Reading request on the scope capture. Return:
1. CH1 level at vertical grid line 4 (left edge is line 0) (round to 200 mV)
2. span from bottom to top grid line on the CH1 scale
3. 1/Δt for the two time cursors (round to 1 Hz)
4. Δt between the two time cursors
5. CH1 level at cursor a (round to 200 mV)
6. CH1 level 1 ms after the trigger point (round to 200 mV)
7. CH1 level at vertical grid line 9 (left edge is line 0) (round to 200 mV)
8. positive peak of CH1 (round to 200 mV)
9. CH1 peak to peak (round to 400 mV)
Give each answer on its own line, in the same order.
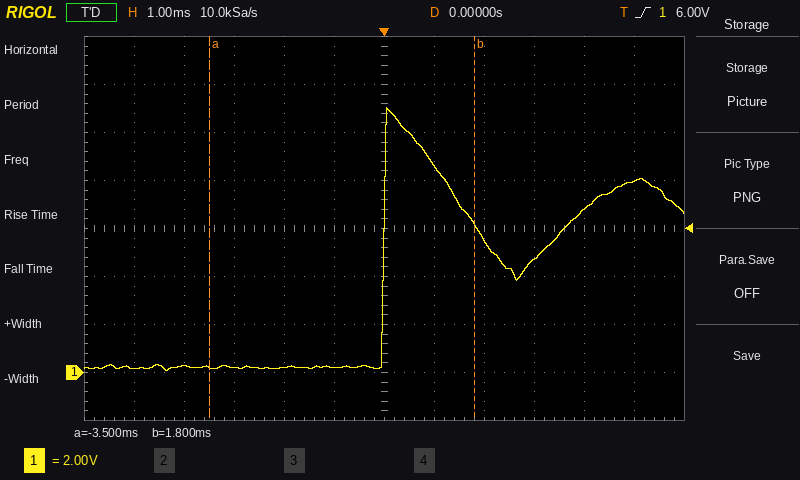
200 mV
16 V
189 Hz
5.3 ms
200 mV
8.6 V
4.8 V
11.0 V
10.8 V
